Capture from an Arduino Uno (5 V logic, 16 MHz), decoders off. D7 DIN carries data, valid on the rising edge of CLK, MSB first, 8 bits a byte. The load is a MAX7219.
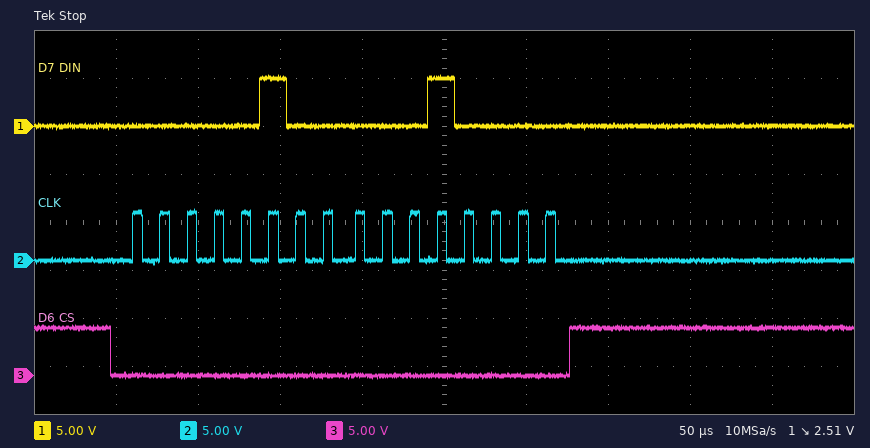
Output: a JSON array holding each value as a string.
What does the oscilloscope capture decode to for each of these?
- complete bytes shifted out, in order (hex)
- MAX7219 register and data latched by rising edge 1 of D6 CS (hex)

["0x04 0x10", "register 0x4, data 0x10"]
